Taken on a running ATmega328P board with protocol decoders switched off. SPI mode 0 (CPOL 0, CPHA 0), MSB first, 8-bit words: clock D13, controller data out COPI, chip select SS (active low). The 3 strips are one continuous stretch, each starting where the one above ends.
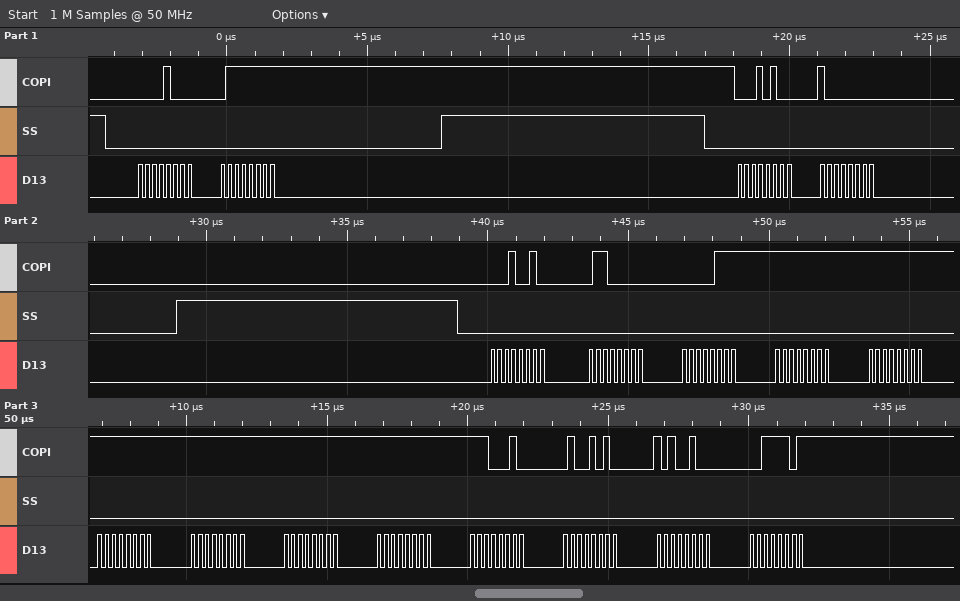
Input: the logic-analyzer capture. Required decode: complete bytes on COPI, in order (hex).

0x08 0x7F 0x14 0x80 0x12 0x60 0x07 0xFF 0xFF 0xFF 0xFF 0xFF 0xFF 0xE2 0x4A 0xA4 0x3D
